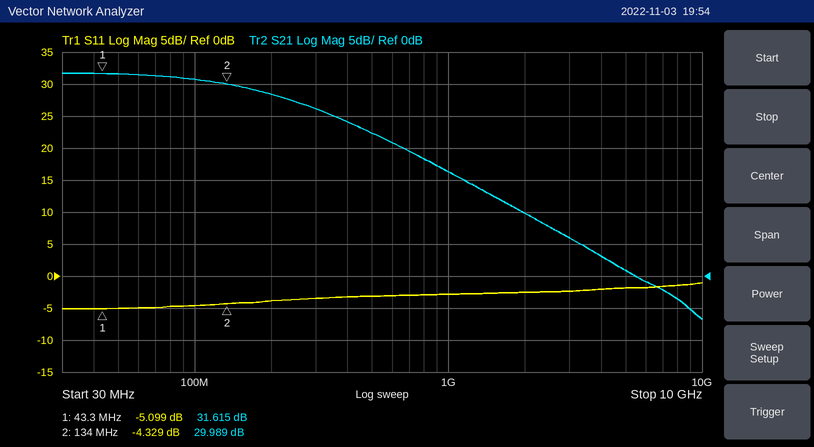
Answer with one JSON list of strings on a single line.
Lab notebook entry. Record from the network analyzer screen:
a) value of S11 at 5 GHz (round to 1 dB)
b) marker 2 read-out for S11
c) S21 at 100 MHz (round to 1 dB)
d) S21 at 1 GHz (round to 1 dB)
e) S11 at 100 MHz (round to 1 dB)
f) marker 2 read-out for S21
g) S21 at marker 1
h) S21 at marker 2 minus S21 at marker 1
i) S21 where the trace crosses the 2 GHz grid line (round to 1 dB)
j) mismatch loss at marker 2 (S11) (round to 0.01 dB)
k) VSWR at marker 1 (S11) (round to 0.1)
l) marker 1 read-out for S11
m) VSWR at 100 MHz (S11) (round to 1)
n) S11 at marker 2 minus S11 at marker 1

["-2 dB", "-4.329 dB", "31 dB", "16 dB", "-5 dB", "29.989 dB", "31.615 dB", "-1.626 dB", "10 dB", "2.00 dB", "3.5", "-5.099 dB", "4", "0.770 dB"]
